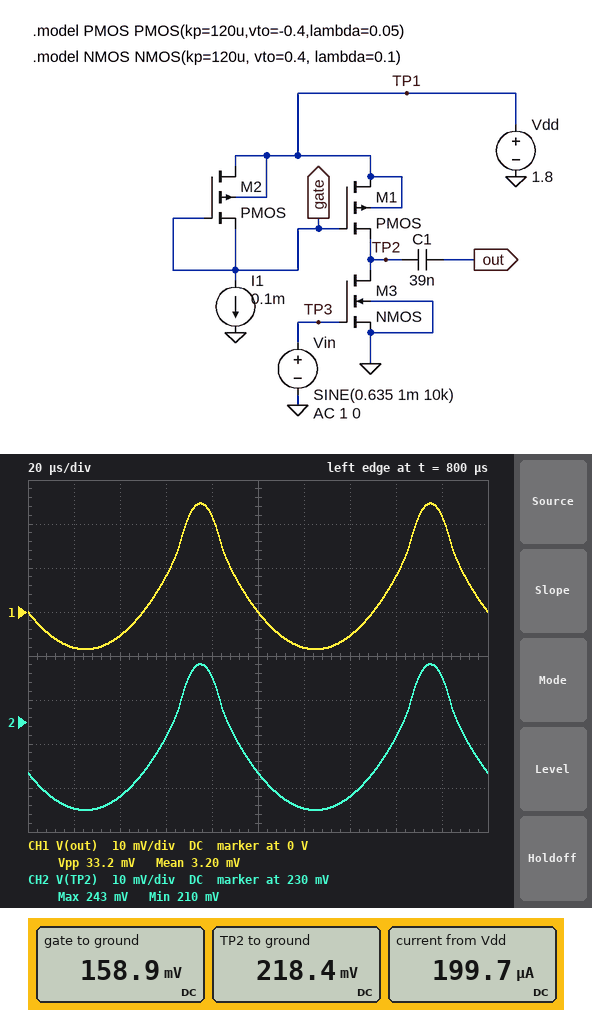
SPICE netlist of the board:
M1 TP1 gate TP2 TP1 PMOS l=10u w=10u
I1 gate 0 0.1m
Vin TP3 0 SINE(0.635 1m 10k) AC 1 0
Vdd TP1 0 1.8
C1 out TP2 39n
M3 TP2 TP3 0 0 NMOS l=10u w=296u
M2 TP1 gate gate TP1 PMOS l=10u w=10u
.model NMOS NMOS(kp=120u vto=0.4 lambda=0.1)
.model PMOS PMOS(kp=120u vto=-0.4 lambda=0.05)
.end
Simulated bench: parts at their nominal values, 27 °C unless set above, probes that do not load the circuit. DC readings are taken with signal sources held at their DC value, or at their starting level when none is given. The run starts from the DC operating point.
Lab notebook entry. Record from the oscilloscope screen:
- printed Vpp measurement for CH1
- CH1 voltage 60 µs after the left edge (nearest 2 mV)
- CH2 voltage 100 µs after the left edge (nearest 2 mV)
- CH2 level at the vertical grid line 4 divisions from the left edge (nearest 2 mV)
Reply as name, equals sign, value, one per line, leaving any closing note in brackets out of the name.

printed Vpp measurement for CH1 = 33.2 mV
CH1 voltage 60 µs after the left edge = 8 mV
CH2 voltage 100 µs after the left edge = 218 mV
CH2 level at the vertical grid line 4 divisions from the left edge = 240 mV
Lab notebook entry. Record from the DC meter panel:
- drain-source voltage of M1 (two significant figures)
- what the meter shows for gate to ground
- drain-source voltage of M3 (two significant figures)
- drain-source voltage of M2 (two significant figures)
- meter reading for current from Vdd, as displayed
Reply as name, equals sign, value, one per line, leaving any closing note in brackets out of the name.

drain-source voltage of M1 = 1.6 V
what the meter shows for gate to ground = 158.9 mV
drain-source voltage of M3 = 220 mV
drain-source voltage of M2 = 1.6 V
meter reading for current from Vdd, as displayed = 199.7 µA
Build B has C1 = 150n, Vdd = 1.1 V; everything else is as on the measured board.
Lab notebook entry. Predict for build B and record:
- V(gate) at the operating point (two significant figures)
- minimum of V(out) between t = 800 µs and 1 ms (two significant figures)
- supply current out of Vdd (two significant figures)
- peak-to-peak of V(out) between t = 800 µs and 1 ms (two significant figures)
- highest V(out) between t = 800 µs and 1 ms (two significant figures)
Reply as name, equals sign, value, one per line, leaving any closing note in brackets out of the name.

V(gate) at the operating point = -540 mV
minimum of V(out) between t = 800 µs and 1 ms = -1.9 mV
supply current out of Vdd = 190 µA
peak-to-peak of V(out) between t = 800 µs and 1 ms = 3.9 mV
highest V(out) between t = 800 µs and 1 ms = 2.0 mV
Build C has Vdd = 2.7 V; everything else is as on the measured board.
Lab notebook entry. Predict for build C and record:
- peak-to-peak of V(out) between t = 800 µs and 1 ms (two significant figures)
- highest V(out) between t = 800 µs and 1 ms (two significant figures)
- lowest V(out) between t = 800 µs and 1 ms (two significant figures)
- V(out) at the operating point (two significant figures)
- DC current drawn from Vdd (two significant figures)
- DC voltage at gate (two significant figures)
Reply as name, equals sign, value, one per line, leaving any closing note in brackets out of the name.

peak-to-peak of V(out) between t = 800 µs and 1 ms = 120 mV
highest V(out) between t = 800 µs and 1 ms = 61 mV
lowest V(out) between t = 800 µs and 1 ms = -60 mV
V(out) at the operating point = 470 mV
DC current drawn from Vdd = 200 µA
DC voltage at gate = 1.1 V
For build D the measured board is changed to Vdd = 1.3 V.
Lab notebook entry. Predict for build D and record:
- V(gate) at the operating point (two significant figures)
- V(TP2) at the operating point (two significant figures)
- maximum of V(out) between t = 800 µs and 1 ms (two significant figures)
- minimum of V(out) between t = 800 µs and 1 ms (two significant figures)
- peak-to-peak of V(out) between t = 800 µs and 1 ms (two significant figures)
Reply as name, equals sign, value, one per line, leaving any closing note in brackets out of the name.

V(gate) at the operating point = -340 mV
V(TP2) at the operating point = 190 mV
maximum of V(out) between t = 800 µs and 1 ms = 3.8 mV
minimum of V(out) between t = 800 µs and 1 ms = -3.5 mV
peak-to-peak of V(out) between t = 800 µs and 1 ms = 7.3 mV
